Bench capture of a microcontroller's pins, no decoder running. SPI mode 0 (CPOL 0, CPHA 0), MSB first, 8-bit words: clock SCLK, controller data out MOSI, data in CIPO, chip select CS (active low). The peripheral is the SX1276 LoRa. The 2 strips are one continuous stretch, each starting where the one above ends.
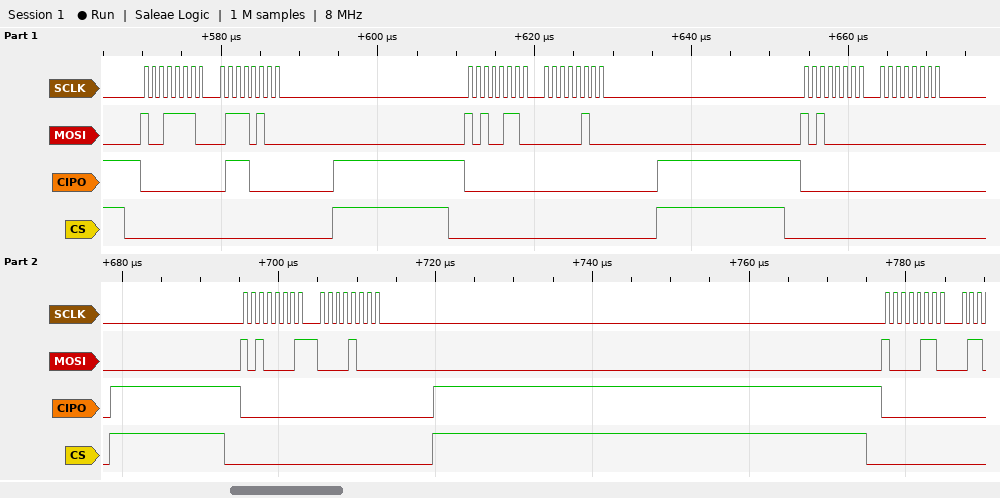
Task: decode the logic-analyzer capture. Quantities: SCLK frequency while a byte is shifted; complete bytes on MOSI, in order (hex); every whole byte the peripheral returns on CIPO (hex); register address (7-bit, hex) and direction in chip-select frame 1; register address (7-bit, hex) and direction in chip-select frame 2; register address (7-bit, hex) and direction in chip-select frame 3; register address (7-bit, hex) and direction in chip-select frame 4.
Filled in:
1 MHz
0x9E 0x74 0xA6 0x04 0xA0 0x00 0xA1 0x08 0x86
0x00 0x70 0x00 0x00 0x00 0x00 0x00 0x00 0x00
0x1E write
0x26 write
0x20 write
0x21 write
